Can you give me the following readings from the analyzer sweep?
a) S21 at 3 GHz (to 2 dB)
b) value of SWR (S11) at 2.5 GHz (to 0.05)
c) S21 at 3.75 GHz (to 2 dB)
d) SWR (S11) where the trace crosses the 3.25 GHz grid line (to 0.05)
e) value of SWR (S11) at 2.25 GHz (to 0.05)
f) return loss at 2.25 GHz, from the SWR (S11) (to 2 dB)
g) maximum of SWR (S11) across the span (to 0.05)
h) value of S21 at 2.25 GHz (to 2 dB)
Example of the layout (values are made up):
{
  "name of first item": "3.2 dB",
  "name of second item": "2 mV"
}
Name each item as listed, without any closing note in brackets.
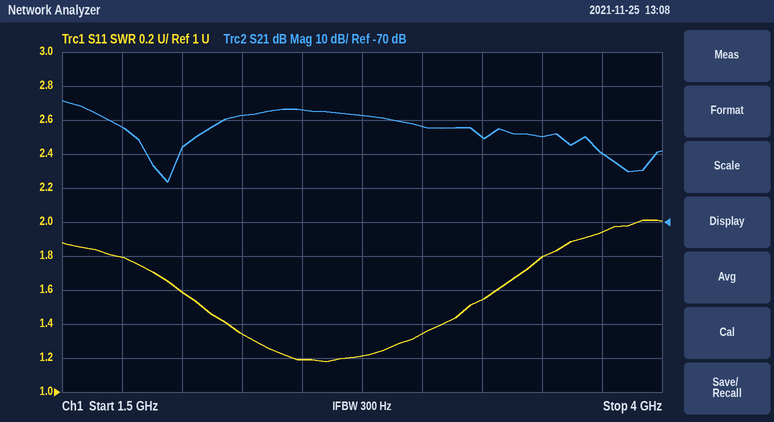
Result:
{
  "S21 at 3 GHz": "-42 dB",
  "value of SWR (S11) at 2.5 GHz": "1.20",
  "S21 at 3.75 GHz": "-50 dB",
  "SWR (S11) where the trace crosses the 3.25 GHz grid line": "1.55",
  "value of SWR (S11) at 2.25 GHz": "1.35",
  "return loss at 2.25 GHz, from the SWR (S11)": "16 dB",
  "maximum of SWR (S11) across the span": "2.00",
  "value of S21 at 2.25 GHz": "-38 dB"
}
